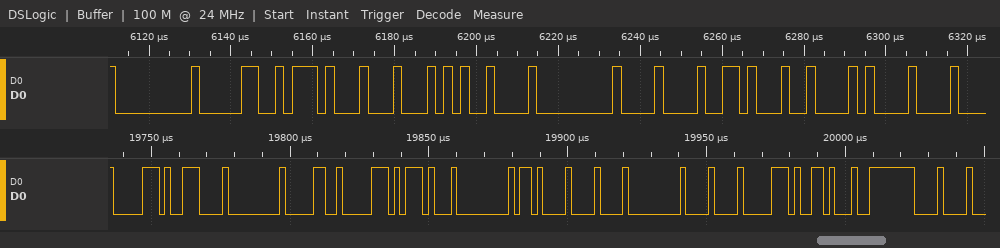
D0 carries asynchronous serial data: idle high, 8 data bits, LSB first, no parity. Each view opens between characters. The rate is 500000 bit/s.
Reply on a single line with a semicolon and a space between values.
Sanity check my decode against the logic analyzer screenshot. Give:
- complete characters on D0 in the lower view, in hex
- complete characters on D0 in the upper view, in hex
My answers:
70, 0E, 00, 30, 70, 17, 00, 0B, 08, 00, 08, 70, 16, FE, 08; 00, 30, 17, 44, 09, 00, 08, 16, 42, 08
